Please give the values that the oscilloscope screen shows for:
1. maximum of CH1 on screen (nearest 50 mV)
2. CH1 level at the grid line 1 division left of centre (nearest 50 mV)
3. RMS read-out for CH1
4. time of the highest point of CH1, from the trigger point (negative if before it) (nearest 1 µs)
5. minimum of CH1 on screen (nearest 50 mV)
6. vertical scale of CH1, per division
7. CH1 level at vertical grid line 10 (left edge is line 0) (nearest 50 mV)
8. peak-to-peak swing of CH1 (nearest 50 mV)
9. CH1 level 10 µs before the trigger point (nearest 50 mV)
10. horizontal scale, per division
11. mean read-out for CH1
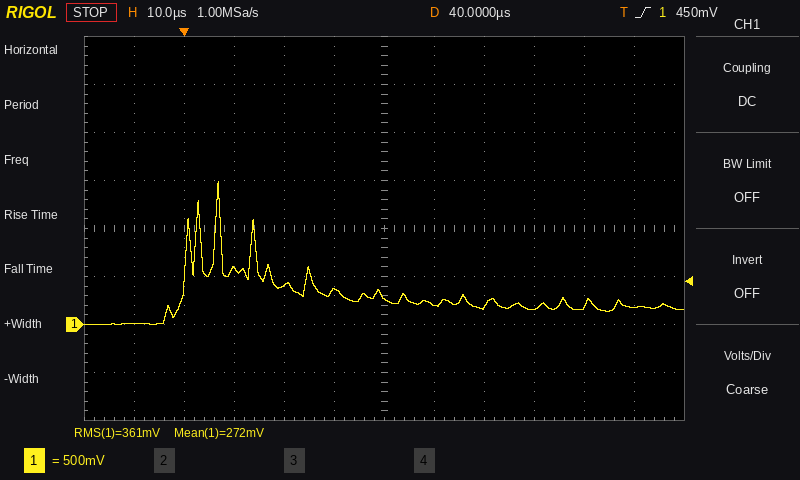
1.50 V
350 mV
361 mV
+7 µs
0 mV
500 mV
200 mV
1.50 V
0 mV
10 µs
272 mV
